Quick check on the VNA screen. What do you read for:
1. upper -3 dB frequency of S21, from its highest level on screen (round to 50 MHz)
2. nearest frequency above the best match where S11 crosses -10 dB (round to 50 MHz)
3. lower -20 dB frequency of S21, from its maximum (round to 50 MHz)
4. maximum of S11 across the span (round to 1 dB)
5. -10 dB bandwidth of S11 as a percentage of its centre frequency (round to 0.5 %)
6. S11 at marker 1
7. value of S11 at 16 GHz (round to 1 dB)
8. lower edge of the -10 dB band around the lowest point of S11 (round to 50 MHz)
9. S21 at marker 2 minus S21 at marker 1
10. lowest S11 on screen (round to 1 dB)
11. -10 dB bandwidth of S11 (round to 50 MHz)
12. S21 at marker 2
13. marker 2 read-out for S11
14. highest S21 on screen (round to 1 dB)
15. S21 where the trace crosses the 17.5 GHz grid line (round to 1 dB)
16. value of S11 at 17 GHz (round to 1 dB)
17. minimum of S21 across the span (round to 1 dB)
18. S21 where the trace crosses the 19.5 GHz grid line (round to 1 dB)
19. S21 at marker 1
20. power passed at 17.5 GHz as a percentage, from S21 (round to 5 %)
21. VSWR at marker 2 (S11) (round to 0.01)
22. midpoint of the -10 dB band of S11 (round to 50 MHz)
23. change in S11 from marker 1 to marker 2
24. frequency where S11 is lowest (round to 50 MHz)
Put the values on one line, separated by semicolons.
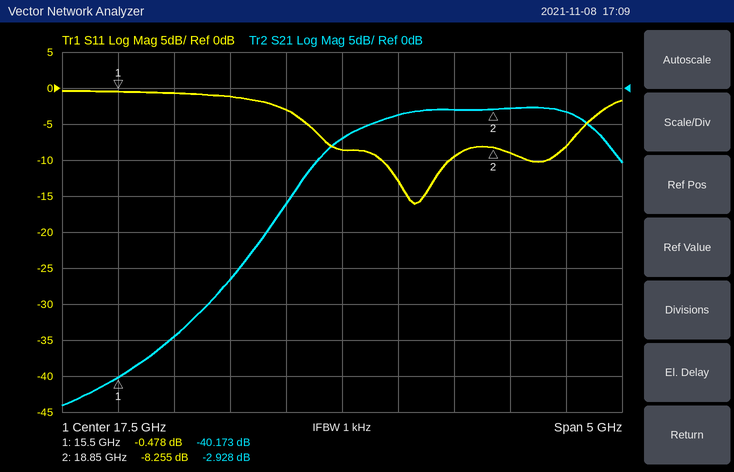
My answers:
19.75 GHz; 18.45 GHz; 16.70 GHz; 0 dB; 3.5 %; -0.478 dB; -1 dB; 17.85 GHz; 37.245 dB; -16 dB; 600 MHz; -2.928 dB; -8.255 dB; -3 dB; -7 dB; -3 dB; -44 dB; -3 dB; -40.173 dB; 20 %; 2.26; 18.15 GHz; -7.777 dB; 18.15 GHz
